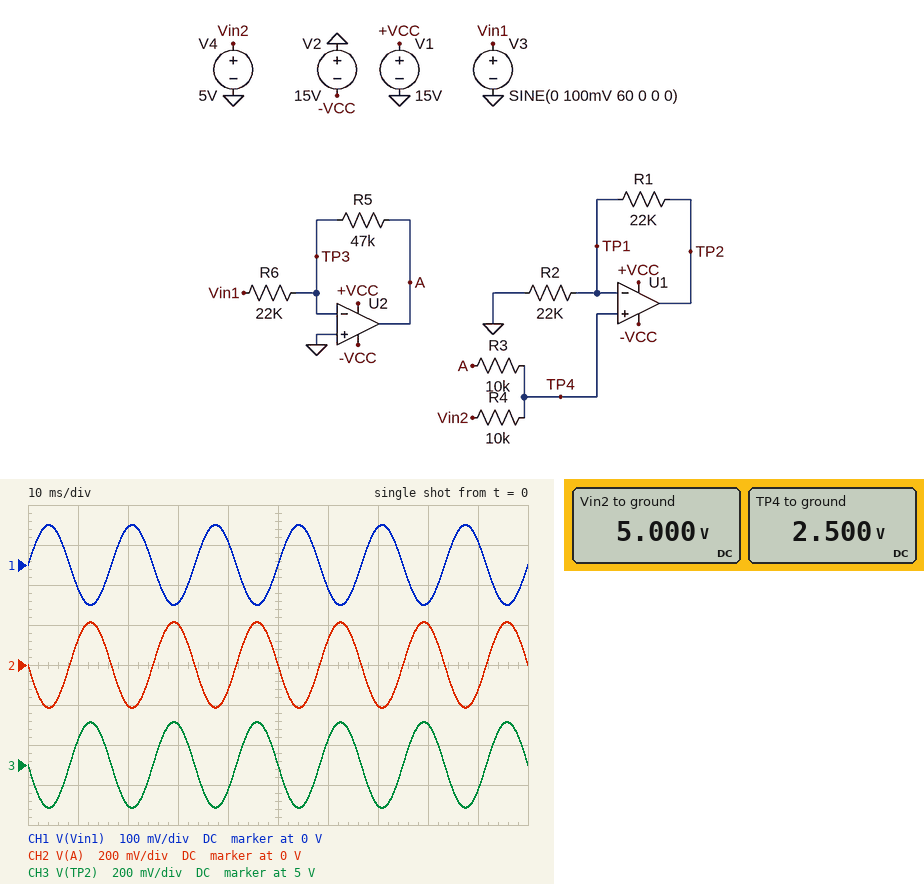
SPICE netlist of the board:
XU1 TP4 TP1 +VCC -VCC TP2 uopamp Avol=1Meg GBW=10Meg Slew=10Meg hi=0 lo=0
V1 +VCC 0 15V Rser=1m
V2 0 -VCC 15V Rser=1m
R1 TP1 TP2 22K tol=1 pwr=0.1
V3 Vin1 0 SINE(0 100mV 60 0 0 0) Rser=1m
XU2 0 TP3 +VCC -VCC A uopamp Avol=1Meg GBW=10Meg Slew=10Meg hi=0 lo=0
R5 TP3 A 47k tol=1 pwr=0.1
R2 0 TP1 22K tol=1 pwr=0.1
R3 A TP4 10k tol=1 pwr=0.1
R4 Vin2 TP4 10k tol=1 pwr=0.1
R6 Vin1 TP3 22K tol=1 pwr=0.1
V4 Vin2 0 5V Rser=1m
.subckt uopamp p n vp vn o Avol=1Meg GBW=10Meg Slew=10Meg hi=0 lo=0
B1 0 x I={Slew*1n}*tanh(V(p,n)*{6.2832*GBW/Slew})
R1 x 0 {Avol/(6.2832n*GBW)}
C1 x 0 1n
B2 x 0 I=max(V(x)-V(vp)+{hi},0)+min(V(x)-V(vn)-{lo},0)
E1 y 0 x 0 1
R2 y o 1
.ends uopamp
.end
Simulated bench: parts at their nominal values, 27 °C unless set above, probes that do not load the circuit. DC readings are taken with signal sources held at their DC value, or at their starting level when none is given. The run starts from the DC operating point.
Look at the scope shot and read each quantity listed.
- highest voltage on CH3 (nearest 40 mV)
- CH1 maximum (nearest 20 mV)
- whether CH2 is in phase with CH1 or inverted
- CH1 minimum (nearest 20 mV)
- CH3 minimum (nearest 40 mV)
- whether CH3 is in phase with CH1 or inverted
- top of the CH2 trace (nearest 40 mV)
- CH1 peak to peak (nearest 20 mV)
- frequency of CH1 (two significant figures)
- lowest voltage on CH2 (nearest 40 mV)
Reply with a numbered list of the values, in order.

1. 5.20 V
2. 100 mV
3. inverted
4. -100 mV
5. 4.80 V
6. inverted
7. 200 mV
8. 200 mV
9. 60 Hz
10. -200 mV
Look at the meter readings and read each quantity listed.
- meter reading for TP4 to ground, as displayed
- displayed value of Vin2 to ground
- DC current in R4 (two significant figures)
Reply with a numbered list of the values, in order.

1. 2.500 V
2. 5.000 V
3. 250 µA
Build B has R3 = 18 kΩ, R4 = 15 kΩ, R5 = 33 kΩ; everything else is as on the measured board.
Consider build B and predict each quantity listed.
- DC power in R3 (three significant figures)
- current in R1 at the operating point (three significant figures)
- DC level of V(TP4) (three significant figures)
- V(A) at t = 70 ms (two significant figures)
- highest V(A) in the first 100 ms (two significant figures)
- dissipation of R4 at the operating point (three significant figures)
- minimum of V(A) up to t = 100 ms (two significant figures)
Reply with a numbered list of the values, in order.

1. 413 µW
2. 124 µA
3. 2.73 V
4. -140 mV
5. 150 mV
6. 344 µW
7. -150 mV
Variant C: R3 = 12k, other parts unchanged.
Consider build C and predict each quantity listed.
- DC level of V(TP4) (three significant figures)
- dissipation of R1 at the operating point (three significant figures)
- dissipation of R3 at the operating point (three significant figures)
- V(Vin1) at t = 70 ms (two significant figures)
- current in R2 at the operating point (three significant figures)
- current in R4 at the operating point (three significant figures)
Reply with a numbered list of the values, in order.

1. 2.73 V
2. 338 µW
3. 620 µW
4. 95 mV
5. 124 µA
6. 227 µA
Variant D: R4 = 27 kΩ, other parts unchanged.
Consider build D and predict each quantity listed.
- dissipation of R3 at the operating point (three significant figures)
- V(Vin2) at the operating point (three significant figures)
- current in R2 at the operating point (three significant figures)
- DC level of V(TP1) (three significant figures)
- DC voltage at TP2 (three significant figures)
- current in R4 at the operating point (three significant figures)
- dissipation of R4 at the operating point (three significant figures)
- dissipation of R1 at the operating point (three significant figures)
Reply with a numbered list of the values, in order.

1. 183 µW
2. 5.00 V
3. 61.4 µA
4. 1.35 V
5. 2.70 V
6. 135 µA
7. 493 µW
8. 83.0 µW
